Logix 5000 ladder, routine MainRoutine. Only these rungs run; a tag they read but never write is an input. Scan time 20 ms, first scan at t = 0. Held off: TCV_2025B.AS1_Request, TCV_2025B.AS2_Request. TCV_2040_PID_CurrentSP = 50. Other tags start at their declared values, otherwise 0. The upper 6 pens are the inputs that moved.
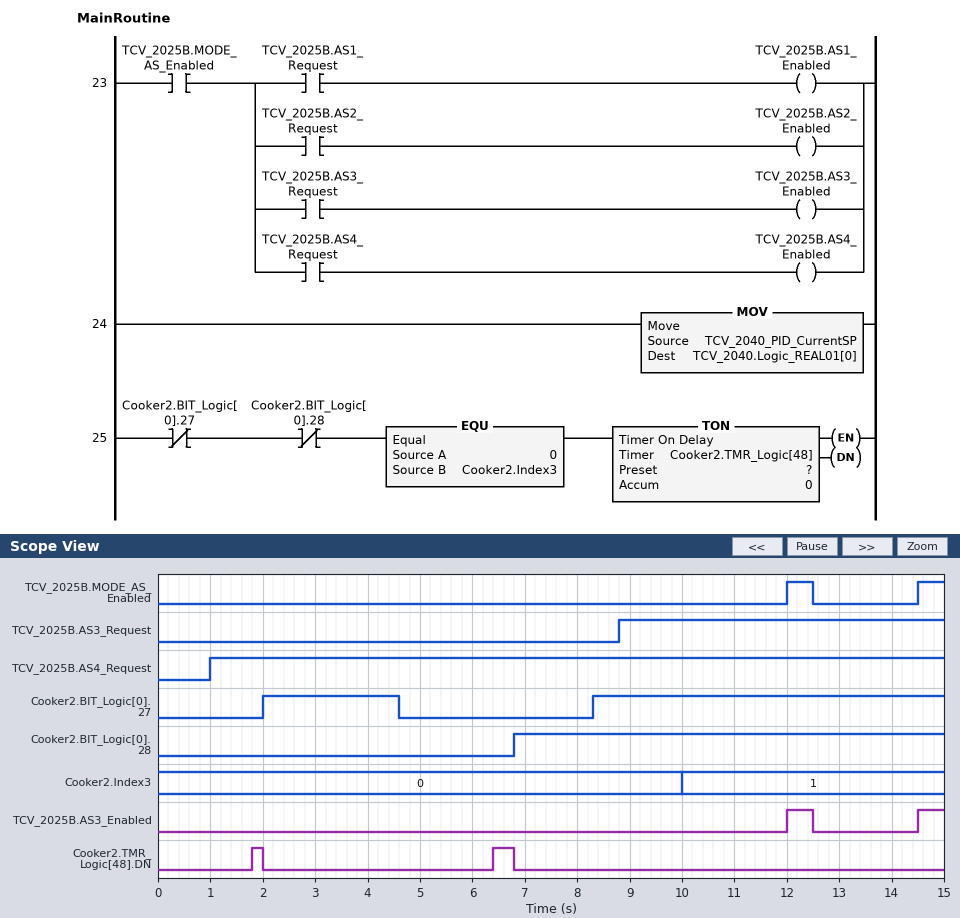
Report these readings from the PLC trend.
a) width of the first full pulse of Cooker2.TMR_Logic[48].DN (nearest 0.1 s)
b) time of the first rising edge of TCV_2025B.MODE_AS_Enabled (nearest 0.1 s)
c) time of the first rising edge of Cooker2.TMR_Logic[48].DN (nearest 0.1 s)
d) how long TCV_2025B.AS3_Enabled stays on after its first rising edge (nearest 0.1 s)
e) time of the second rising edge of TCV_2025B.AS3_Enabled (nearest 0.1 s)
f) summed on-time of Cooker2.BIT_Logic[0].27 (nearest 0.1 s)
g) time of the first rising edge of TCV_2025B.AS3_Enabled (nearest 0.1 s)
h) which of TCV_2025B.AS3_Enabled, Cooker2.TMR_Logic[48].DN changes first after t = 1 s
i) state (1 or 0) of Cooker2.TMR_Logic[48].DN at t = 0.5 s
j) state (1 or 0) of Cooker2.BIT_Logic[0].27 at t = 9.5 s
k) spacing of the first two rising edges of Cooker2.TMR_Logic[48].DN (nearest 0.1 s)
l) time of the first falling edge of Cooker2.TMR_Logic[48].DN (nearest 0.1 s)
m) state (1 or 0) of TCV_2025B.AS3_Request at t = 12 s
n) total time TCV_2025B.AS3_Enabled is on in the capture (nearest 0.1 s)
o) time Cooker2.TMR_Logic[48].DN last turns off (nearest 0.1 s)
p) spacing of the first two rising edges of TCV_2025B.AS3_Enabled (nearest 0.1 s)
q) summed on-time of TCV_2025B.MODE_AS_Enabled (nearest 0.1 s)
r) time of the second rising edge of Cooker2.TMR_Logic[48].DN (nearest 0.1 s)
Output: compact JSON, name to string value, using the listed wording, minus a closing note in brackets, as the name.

{"width of the first full pulse of Cooker2.TMR_Logic[48].DN": "0.2 s", "time of the first rising edge of TCV_2025B.MODE_AS_Enabled": "12.0 s", "time of the first rising edge of Cooker2.TMR_Logic[48].DN": "1.8 s", "how long TCV_2025B.AS3_Enabled stays on after its first rising edge": "0.5 s", "time of the second rising edge of TCV_2025B.AS3_Enabled": "14.5 s", "summed on-time of Cooker2.BIT_Logic[0].27": "9.3 s", "time of the first rising edge of TCV_2025B.AS3_Enabled": "12.0 s", "which of TCV_2025B.AS3_Enabled, Cooker2.TMR_Logic[48].DN changes first after t = 1 s": "Cooker2.TMR_Logic[48].DN", "state (1 or 0) of Cooker2.TMR_Logic[48].DN at t = 0.5 s": "0", "state (1 or 0) of Cooker2.BIT_Logic[0].27 at t = 9.5 s": "1", "spacing of the first two rising edges of Cooker2.TMR_Logic[48].DN": "4.6 s", "time of the first falling edge of Cooker2.TMR_Logic[48].DN": "2.0 s", "state (1 or 0) of TCV_2025B.AS3_Request at t = 12 s": "1", "total time TCV_2025B.AS3_Enabled is on in the capture": "1.0 s", "time Cooker2.TMR_Logic[48].DN last turns off": "6.8 s", "spacing of the first two rising edges of TCV_2025B.AS3_Enabled": "2.5 s", "summed on-time of TCV_2025B.MODE_AS_Enabled": "1.0 s", "time of the second rising edge of Cooker2.TMR_Logic[48].DN": "6.4 s"}
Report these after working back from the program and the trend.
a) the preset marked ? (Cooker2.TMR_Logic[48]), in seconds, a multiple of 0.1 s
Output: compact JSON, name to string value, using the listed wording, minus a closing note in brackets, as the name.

{"the preset marked ? (Cooker2.TMR_Logic[48]), in seconds, a multiple of 0.1 s": "1.8 s"}
